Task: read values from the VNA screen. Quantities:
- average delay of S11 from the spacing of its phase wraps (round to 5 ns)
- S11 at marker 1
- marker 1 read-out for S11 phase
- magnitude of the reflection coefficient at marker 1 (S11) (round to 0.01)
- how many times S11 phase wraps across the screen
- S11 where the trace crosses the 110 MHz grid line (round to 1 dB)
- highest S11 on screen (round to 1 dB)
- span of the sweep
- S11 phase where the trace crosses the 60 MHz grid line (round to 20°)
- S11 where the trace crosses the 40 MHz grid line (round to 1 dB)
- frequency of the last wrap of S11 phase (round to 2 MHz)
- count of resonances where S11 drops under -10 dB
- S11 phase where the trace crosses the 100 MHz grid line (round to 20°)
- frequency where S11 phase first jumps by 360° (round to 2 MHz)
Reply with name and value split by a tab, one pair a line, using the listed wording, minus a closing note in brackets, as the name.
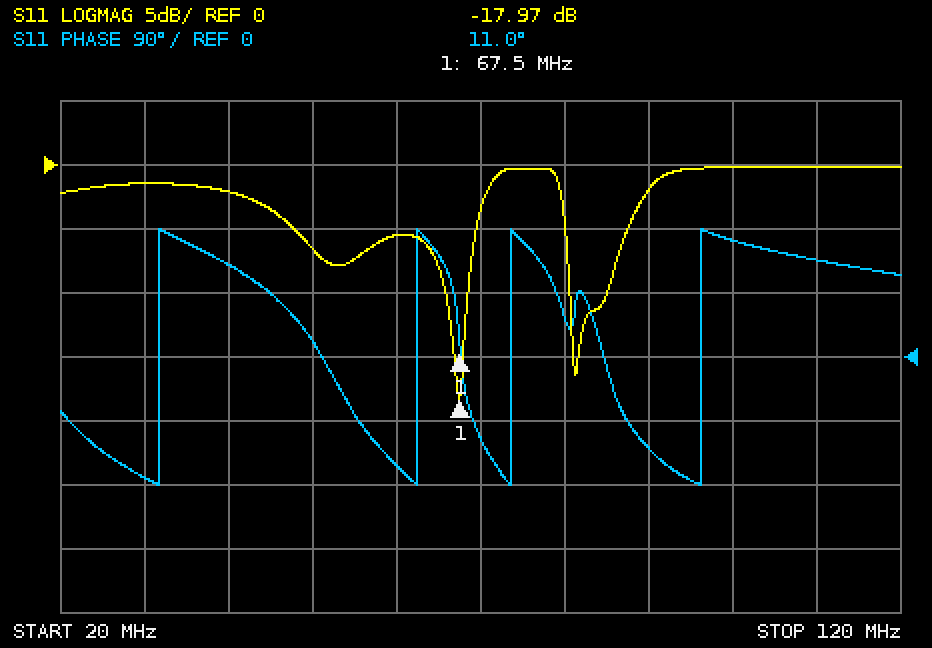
average delay of S11 from the spacing of its phase wraps	45 ns
S11 at marker 1	-17.97 dB
marker 1 read-out for S11 phase	11.0°
magnitude of the reflection coefficient at marker 1 (S11)	0.13
how many times S11 phase wraps across the screen	4
S11 where the trace crosses the 110 MHz grid line	0 dB
highest S11 on screen	0 dB
span of the sweep	100 MHz
S11 phase where the trace crosses the 60 MHz grid line	-160°
S11 where the trace crosses the 40 MHz grid line	-2 dB
frequency of the last wrap of S11 phase	96 MHz
count of resonances where S11 drops under -10 dB	2
S11 phase where the trace crosses the 100 MHz grid line	160°
frequency where S11 phase first jumps by 360°	32 MHz
